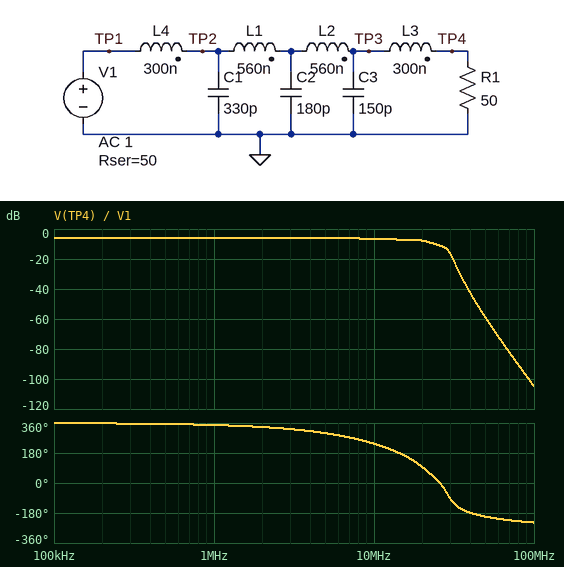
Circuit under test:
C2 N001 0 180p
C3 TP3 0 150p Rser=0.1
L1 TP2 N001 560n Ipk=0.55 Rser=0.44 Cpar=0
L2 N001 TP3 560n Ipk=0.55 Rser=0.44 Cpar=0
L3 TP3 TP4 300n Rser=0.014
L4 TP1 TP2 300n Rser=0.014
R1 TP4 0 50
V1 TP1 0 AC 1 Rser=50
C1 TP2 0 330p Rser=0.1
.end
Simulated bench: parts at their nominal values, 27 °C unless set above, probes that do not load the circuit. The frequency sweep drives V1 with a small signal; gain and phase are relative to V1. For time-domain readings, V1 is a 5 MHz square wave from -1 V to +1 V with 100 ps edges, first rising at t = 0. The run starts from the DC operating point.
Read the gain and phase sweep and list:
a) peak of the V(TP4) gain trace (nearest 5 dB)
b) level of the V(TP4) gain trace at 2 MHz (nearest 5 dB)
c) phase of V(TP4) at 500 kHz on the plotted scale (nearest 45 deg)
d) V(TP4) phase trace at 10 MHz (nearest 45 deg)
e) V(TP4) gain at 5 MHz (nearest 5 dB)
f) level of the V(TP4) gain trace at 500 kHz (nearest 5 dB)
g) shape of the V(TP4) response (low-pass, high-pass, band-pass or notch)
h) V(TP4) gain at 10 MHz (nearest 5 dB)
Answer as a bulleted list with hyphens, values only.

- -5 dB
- -5 dB
- 360 deg
- 225 deg
- -5 dB
- -5 dB
- low-pass
- -5 dB
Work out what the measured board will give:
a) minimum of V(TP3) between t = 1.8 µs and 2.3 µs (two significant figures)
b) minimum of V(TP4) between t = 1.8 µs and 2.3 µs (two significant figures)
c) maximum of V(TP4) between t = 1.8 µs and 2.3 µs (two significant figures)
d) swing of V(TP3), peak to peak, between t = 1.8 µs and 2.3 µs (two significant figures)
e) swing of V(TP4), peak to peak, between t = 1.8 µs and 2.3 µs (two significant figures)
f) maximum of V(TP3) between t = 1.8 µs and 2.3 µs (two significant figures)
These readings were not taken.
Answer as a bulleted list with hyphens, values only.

- -670 mV
- -600 mV
- 600 mV
- 1.3 V
- 1.2 V
- 670 mV
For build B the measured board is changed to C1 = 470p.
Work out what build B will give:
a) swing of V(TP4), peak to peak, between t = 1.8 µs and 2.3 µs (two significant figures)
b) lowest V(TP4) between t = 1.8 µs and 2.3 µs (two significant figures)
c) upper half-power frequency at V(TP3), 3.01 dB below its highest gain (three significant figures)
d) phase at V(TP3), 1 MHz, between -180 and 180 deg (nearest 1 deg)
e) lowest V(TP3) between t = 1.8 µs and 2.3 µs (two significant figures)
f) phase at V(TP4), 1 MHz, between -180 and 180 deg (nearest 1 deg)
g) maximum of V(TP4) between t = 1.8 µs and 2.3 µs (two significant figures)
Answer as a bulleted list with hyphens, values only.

- 1.1 V
- -530 mV
- 20.9 MHz
- -11 deg
- -570 mV
- -13 deg
- 530 mV
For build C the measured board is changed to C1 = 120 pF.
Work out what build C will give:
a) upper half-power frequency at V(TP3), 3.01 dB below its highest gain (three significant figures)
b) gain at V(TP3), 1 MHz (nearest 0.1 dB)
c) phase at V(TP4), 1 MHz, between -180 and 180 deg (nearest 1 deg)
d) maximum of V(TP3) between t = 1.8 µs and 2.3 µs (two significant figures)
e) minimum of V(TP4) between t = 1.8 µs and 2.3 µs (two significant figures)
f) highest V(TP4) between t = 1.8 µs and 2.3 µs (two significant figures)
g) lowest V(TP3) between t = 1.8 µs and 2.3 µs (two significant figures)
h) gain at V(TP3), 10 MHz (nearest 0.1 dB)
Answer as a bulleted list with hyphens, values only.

- 32.5 MHz
- -6.1 dB
- -10 deg
- 760 mV
- -650 mV
- 650 mV
- -760 mV
- -5.6 dB
